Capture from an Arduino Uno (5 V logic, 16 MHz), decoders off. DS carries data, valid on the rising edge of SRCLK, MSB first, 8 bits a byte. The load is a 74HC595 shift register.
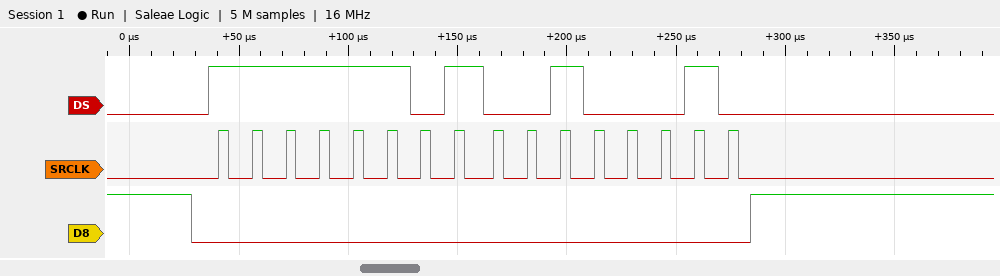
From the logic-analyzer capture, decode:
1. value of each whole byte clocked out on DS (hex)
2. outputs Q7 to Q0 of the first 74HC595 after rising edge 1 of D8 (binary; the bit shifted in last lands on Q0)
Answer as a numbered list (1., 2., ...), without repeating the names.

1. FD 22
2. 00100010
